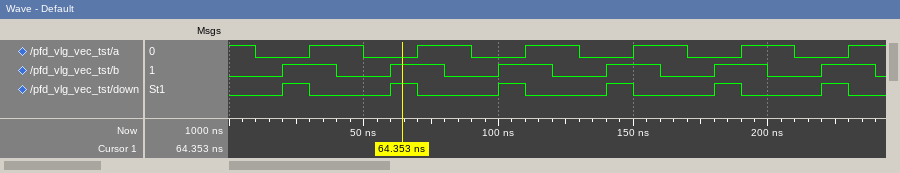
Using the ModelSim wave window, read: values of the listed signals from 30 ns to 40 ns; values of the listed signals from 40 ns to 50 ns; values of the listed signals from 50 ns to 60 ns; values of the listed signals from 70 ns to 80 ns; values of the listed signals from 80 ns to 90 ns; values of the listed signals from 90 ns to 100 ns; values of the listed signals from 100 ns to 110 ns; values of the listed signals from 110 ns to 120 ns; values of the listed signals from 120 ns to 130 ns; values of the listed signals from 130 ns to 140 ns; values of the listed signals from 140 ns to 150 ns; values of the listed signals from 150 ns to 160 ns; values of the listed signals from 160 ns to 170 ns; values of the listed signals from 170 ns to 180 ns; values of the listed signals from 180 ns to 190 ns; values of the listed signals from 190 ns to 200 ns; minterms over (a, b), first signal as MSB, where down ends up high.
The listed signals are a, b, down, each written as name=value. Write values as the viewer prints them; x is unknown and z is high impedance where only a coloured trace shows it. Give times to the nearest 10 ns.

a=1, b=1, down=0
a=1, b=0, down=0
a=0, b=0, down=0
a=1, b=1, down=0
a=1, b=0, down=0
a=0, b=0, down=0
a=0, b=1, down=1
a=1, b=1, down=0
a=1, b=0, down=0
a=0, b=0, down=0
a=0, b=1, down=1
a=1, b=1, down=0
a=1, b=0, down=0
a=0, b=0, down=0
a=0, b=1, down=1
a=1, b=1, down=0
1
